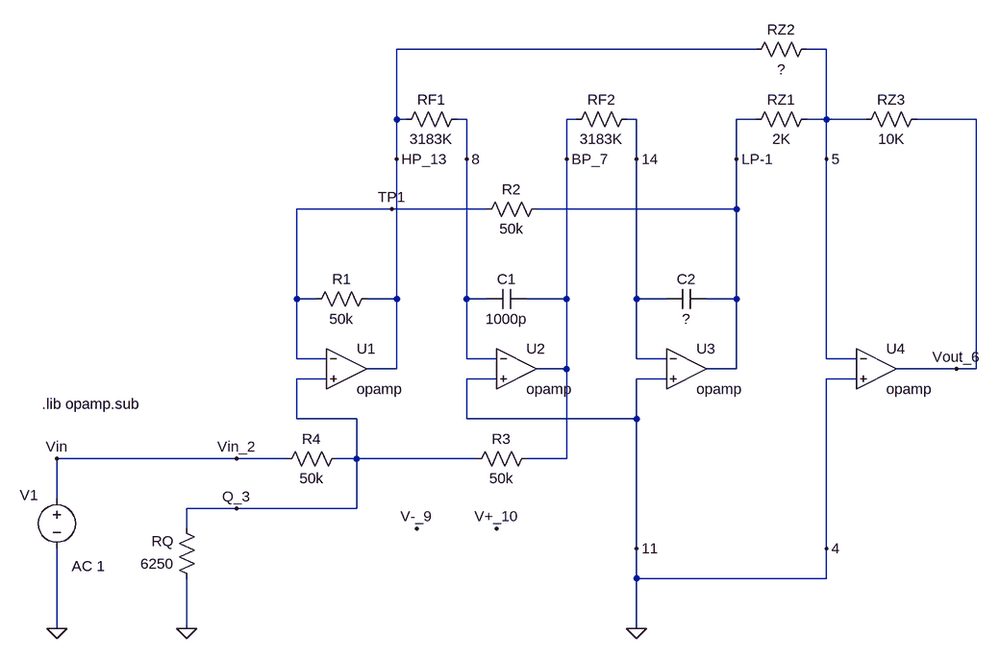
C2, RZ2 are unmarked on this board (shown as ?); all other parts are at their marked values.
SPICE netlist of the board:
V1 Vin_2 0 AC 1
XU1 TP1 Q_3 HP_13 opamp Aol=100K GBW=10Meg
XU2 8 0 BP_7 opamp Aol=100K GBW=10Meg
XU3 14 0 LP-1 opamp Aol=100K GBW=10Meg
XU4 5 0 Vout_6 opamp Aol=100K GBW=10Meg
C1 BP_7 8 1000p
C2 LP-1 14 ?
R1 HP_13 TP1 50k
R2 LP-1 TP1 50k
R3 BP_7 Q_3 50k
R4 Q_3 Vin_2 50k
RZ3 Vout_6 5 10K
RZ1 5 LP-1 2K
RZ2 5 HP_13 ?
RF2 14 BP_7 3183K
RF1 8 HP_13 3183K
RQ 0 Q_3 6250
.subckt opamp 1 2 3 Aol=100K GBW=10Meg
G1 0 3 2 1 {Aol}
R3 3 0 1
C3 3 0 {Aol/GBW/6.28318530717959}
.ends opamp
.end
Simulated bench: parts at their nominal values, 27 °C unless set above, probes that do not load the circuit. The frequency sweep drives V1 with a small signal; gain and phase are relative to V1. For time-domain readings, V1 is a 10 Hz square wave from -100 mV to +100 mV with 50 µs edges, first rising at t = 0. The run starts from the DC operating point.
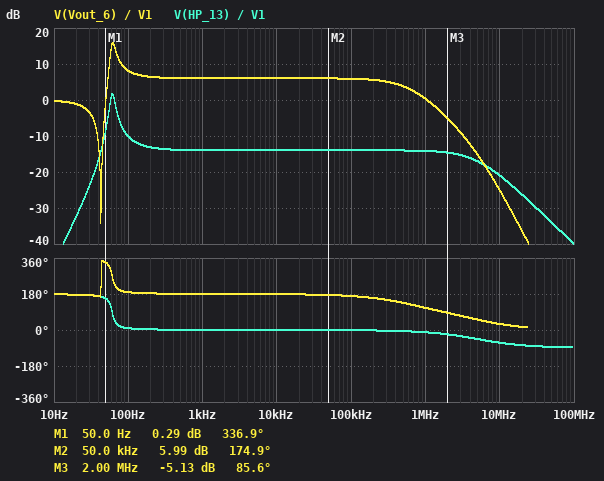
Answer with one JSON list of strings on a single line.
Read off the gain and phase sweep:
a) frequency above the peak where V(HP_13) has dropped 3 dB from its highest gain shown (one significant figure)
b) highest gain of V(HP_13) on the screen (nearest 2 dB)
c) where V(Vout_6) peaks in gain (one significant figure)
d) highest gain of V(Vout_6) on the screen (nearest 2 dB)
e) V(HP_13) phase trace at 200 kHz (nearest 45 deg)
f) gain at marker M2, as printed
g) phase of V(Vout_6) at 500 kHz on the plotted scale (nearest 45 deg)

["70 Hz", "2 dB", "60 Hz", "16 dB", "0 deg", "5.99 dB", "135 deg"]
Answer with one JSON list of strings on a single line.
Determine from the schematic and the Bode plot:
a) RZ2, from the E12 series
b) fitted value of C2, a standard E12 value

["1 kΩ", "680 pF"]
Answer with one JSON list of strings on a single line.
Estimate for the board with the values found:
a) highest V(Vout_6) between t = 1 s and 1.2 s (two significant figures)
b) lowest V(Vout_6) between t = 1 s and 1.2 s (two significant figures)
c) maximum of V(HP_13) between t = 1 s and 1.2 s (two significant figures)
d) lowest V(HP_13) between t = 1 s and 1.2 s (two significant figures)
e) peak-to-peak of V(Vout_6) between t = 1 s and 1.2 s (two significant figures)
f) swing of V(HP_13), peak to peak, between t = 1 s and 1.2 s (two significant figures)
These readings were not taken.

["270 mV", "-270 mV", "33 mV", "-33 mV", "530 mV", "66 mV"]
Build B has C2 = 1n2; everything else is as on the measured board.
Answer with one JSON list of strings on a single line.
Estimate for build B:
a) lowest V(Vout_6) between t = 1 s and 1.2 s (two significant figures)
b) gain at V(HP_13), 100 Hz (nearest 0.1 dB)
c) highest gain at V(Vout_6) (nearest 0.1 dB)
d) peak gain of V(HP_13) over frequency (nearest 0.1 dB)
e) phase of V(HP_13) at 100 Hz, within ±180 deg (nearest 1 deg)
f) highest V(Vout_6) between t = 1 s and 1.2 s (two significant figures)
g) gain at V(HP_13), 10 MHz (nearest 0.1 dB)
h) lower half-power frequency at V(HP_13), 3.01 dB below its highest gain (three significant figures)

["-310 mV", "-12.0 dB", "13.6 dB", "-0.7 dB", "7 deg", "310 mV", "-21.0 dB", "41.8 Hz"]
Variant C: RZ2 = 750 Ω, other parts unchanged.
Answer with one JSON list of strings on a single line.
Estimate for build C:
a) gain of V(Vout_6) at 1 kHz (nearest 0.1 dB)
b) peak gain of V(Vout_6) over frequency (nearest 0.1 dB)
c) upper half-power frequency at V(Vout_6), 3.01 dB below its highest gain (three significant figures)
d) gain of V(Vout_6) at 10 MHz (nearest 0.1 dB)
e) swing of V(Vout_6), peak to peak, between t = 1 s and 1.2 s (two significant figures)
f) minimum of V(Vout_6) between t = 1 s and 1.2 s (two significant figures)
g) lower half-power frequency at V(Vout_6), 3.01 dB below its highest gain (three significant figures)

["8.5 dB", "20.2 dB", "68.4 Hz", "-24.2 dB", "750 mV", "-380 mV", "57.3 Hz"]
